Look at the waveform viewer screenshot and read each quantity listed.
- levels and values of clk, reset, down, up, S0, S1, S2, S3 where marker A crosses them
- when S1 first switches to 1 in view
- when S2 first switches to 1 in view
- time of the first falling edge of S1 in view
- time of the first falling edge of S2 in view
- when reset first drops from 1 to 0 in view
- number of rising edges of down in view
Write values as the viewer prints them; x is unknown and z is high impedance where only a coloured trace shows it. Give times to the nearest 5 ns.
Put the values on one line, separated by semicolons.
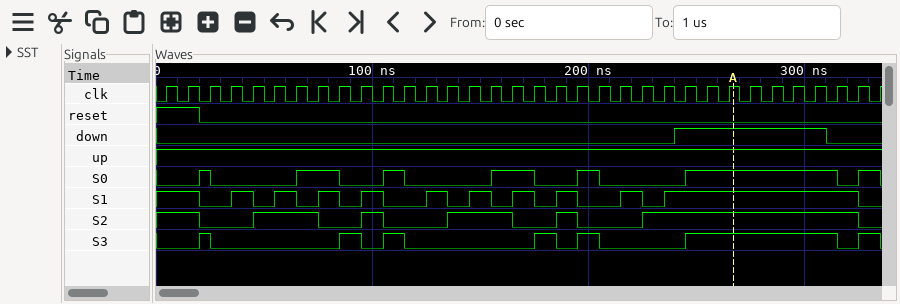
clk=1, reset=0, down=1, up=1, S0=1, S1=1, S2=1, S3=1; 35 ns; 45 ns; 20 ns; 20 ns; 20 ns; 1
